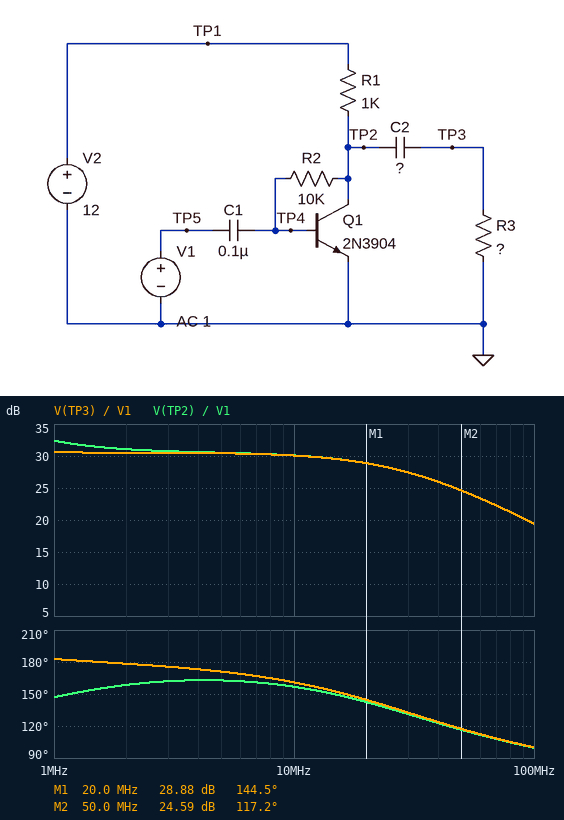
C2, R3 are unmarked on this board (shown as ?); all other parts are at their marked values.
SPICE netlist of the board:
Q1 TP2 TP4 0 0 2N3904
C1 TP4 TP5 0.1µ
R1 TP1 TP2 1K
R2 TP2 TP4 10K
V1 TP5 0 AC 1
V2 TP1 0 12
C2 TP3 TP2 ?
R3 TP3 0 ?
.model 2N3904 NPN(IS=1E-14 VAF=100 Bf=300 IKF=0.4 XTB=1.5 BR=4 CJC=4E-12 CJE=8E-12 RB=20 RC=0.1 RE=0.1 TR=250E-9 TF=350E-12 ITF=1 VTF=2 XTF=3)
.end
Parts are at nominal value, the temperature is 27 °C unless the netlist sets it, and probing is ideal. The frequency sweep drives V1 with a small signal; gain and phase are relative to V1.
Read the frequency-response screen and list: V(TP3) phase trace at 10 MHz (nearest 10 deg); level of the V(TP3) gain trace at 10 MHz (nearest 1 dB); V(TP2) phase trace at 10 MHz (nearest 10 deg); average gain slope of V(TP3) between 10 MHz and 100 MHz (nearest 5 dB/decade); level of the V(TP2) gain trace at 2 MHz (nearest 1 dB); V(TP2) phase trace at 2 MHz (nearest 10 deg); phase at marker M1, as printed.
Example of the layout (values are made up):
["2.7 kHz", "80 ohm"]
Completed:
["160 deg", "30 dB", "160 deg", "-10 dB/decade", "31 dB", "160 deg", "144.5 deg"]
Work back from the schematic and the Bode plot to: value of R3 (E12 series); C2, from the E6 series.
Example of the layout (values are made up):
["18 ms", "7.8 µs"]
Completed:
["100 Ω", "2.2 nF"]
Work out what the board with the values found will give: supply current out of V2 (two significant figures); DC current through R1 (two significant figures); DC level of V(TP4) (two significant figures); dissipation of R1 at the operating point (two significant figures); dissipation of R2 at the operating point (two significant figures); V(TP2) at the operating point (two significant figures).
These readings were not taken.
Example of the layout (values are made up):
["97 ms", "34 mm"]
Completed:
["11 mA", "11 mA", "720 mV", "120 mW", "14 µW", "1.1 V"]
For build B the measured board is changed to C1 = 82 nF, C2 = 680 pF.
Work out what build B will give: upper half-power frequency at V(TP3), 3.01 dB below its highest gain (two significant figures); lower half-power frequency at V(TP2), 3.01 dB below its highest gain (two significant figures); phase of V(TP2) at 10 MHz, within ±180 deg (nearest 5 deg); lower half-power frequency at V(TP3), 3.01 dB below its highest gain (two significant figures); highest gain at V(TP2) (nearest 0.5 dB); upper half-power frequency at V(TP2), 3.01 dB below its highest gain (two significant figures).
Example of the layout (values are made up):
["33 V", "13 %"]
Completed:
["30 MHz", "51 kHz", "150 deg", "200 kHz", "49.5 dB", "310 kHz"]
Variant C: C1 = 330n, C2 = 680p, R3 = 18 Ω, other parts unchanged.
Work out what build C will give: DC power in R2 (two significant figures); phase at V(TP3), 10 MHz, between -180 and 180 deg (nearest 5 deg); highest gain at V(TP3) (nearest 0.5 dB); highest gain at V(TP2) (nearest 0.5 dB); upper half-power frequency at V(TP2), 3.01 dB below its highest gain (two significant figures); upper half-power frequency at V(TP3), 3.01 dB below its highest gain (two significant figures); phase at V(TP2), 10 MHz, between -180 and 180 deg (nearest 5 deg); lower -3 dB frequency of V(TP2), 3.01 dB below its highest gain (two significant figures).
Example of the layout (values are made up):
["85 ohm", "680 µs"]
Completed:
["14 µW", "170 deg", "16.0 dB", "50.0 dB", "280 kHz", "48 MHz", "115 deg", "15 kHz"]
